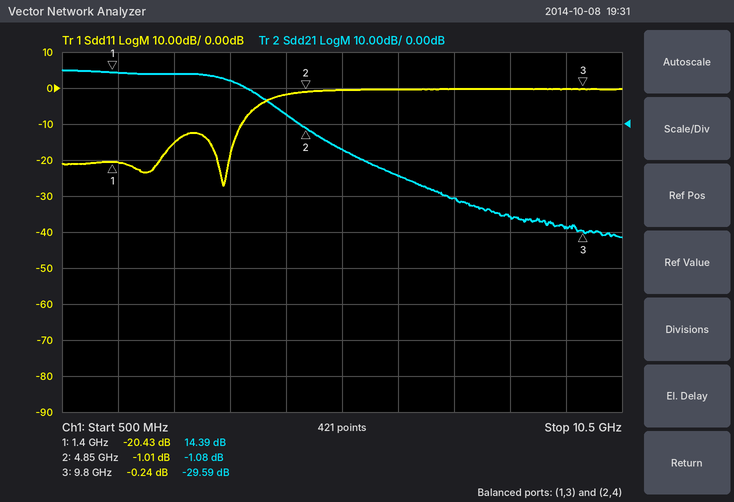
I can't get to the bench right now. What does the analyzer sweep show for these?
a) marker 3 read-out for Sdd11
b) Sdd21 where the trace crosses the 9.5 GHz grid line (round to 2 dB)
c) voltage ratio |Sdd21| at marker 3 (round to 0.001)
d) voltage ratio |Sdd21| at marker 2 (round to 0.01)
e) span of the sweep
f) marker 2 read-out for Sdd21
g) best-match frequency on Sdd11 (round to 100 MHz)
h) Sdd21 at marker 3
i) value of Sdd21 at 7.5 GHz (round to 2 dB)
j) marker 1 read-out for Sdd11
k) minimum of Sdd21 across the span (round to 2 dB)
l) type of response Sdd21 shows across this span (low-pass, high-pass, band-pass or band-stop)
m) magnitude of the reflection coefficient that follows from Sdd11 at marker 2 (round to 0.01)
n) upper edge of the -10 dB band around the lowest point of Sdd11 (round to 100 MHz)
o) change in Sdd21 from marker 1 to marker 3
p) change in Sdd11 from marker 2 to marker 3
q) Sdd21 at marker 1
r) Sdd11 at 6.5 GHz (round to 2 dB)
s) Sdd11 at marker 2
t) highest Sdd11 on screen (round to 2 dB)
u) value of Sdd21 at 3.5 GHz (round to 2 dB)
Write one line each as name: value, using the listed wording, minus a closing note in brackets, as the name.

marker 3 read-out for Sdd11: -0.24 dB
Sdd21 where the trace crosses the 9.5 GHz grid line: -28 dB
voltage ratio |Sdd21| at marker 3: 0.033
voltage ratio |Sdd21| at marker 2: 0.88
span of the sweep: 10 GHz
marker 2 read-out for Sdd21: -1.08 dB
best-match frequency on Sdd11: 3.4 GHz
Sdd21 at marker 3: -29.59 dB
value of Sdd21 at 7.5 GHz: -20 dB
marker 1 read-out for Sdd11: -20.43 dB
minimum of Sdd21 across the span: -32 dB
type of response Sdd21 shows across this span: low-pass
magnitude of the reflection coefficient that follows from Sdd11 at marker 2: 0.89
upper edge of the -10 dB band around the lowest point of Sdd11: 3.7 GHz
change in Sdd21 from marker 1 to marker 3: -43.98 dB
change in Sdd11 from marker 2 to marker 3: 0.77 dB
Sdd21 at marker 1: 14.39 dB
Sdd11 at 6.5 GHz: 0 dB
Sdd11 at marker 2: -1.01 dB
highest Sdd11 on screen: 0 dB
value of Sdd21 at 3.5 GHz: 12 dB
